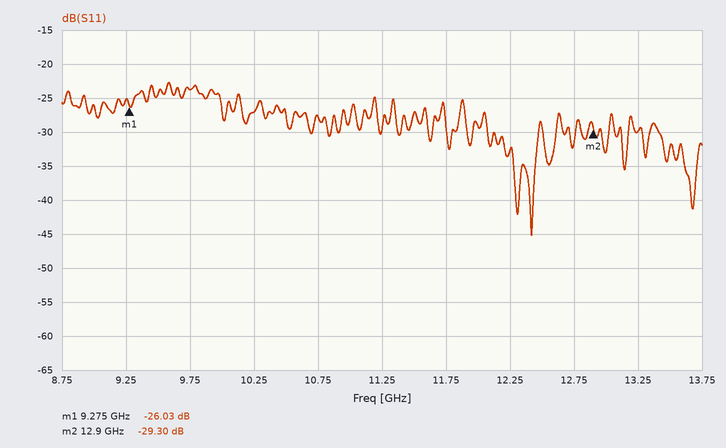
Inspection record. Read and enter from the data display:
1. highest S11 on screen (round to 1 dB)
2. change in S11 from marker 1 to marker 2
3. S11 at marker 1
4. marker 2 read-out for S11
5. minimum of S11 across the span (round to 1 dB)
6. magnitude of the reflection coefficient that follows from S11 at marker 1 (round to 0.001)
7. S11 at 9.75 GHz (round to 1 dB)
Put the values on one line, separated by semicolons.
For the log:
-23 dB; -3.27 dB; -26.03 dB; -29.30 dB; -45 dB; 0.050; -24 dB
